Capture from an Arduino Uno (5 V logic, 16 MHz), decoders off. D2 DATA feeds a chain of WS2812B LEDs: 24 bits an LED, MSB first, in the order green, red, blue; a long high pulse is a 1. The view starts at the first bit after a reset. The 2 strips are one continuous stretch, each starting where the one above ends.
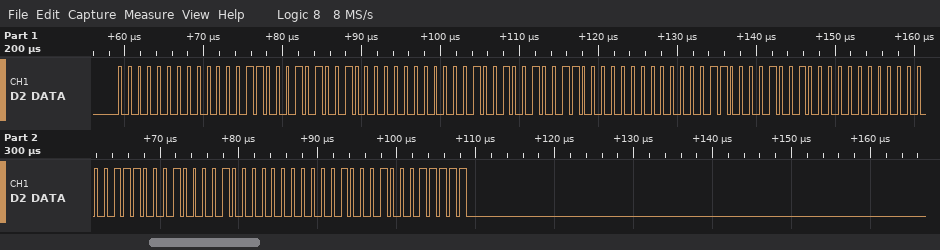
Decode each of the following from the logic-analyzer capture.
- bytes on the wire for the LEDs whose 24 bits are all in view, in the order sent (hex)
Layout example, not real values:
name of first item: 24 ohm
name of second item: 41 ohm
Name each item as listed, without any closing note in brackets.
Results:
bytes on the wire for the LEDs whose 24 bits are all in view, in the order sent: 00 06 29 00 09 26 00 0C 24 00 0E 21 00 11 1F
